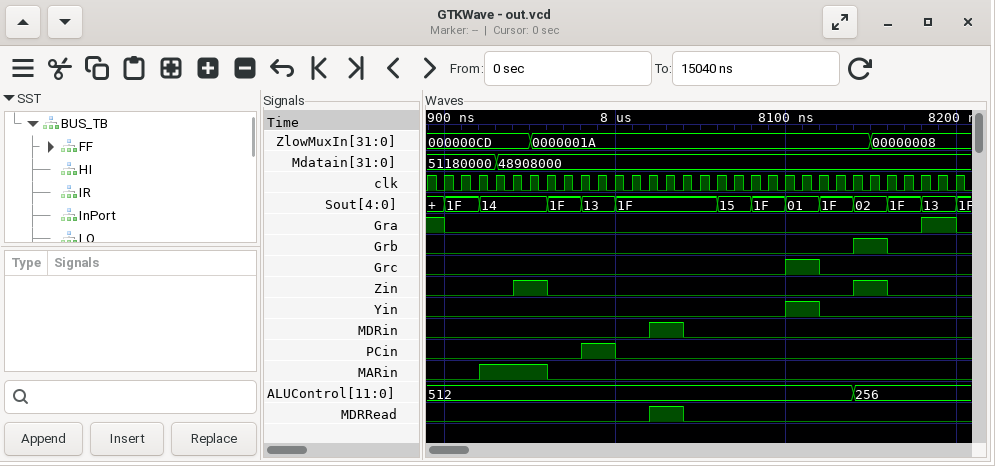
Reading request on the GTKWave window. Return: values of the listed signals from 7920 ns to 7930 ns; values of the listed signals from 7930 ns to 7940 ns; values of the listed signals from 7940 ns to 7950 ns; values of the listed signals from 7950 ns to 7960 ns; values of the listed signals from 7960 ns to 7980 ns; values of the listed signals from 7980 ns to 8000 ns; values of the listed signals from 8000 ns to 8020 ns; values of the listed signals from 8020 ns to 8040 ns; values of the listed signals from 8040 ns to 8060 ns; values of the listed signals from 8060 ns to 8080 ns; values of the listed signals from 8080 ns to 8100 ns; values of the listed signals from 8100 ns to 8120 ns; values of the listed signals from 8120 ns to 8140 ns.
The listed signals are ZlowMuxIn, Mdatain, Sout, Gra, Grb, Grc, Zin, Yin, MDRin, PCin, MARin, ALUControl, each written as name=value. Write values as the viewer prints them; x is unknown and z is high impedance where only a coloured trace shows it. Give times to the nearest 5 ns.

ZlowMuxIn=000000CD, Mdatain=51180000, Sout=14, Gra=0, Grb=0, Grc=0, Zin=0, Yin=0, MDRin=0, PCin=0, MARin=1, ALUControl=512
ZlowMuxIn=000000CD, Mdatain=48908000, Sout=14, Gra=0, Grb=0, Grc=0, Zin=0, Yin=0, MDRin=0, PCin=0, MARin=1, ALUControl=512
ZlowMuxIn=000000CD, Mdatain=48908000, Sout=14, Gra=0, Grb=0, Grc=0, Zin=1, Yin=0, MDRin=0, PCin=0, MARin=1, ALUControl=512
ZlowMuxIn=0000001A, Mdatain=48908000, Sout=14, Gra=0, Grb=0, Grc=0, Zin=1, Yin=0, MDRin=0, PCin=0, MARin=1, ALUControl=512
ZlowMuxIn=0000001A, Mdatain=48908000, Sout=1F, Gra=0, Grb=0, Grc=0, Zin=0, Yin=0, MDRin=0, PCin=0, MARin=0, ALUControl=512
ZlowMuxIn=0000001A, Mdatain=48908000, Sout=13, Gra=0, Grb=0, Grc=0, Zin=0, Yin=0, MDRin=0, PCin=1, MARin=0, ALUControl=512
ZlowMuxIn=0000001A, Mdatain=48908000, Sout=1F, Gra=0, Grb=0, Grc=0, Zin=0, Yin=0, MDRin=0, PCin=0, MARin=0, ALUControl=512
ZlowMuxIn=0000001A, Mdatain=48908000, Sout=1F, Gra=0, Grb=0, Grc=0, Zin=0, Yin=0, MDRin=1, PCin=0, MARin=0, ALUControl=512
ZlowMuxIn=0000001A, Mdatain=48908000, Sout=1F, Gra=0, Grb=0, Grc=0, Zin=0, Yin=0, MDRin=0, PCin=0, MARin=0, ALUControl=512
ZlowMuxIn=0000001A, Mdatain=48908000, Sout=15, Gra=0, Grb=0, Grc=0, Zin=0, Yin=0, MDRin=0, PCin=0, MARin=0, ALUControl=512
ZlowMuxIn=0000001A, Mdatain=48908000, Sout=1F, Gra=0, Grb=0, Grc=0, Zin=0, Yin=0, MDRin=0, PCin=0, MARin=0, ALUControl=512
ZlowMuxIn=0000001A, Mdatain=48908000, Sout=01, Gra=0, Grb=0, Grc=1, Zin=0, Yin=1, MDRin=0, PCin=0, MARin=0, ALUControl=512
ZlowMuxIn=0000001A, Mdatain=48908000, Sout=1F, Gra=0, Grb=0, Grc=0, Zin=0, Yin=0, MDRin=0, PCin=0, MARin=0, ALUControl=512
